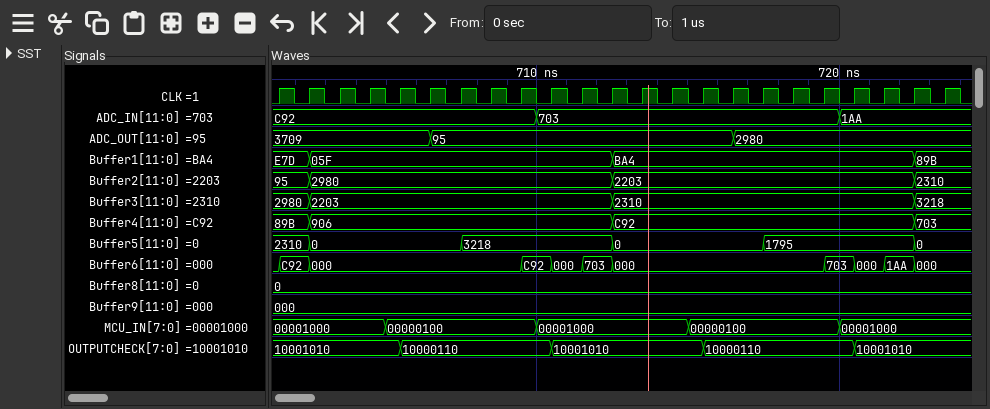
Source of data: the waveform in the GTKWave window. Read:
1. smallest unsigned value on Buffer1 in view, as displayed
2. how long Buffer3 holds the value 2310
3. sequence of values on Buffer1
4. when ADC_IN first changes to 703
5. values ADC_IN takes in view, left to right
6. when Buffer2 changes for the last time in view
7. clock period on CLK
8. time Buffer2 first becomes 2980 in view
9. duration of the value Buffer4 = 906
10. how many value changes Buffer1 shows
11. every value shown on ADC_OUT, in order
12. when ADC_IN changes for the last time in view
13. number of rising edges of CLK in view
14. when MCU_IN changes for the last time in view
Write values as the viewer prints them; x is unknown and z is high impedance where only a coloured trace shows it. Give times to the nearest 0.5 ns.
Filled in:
05F
10 ns
E7D, 05F, BA4, 89B
710 ns
C92, 703, 1AA
722.5 ns
1 ns
702.5 ns
10 ns
3
3709, 95, 2980
720 ns
23
720 ns
